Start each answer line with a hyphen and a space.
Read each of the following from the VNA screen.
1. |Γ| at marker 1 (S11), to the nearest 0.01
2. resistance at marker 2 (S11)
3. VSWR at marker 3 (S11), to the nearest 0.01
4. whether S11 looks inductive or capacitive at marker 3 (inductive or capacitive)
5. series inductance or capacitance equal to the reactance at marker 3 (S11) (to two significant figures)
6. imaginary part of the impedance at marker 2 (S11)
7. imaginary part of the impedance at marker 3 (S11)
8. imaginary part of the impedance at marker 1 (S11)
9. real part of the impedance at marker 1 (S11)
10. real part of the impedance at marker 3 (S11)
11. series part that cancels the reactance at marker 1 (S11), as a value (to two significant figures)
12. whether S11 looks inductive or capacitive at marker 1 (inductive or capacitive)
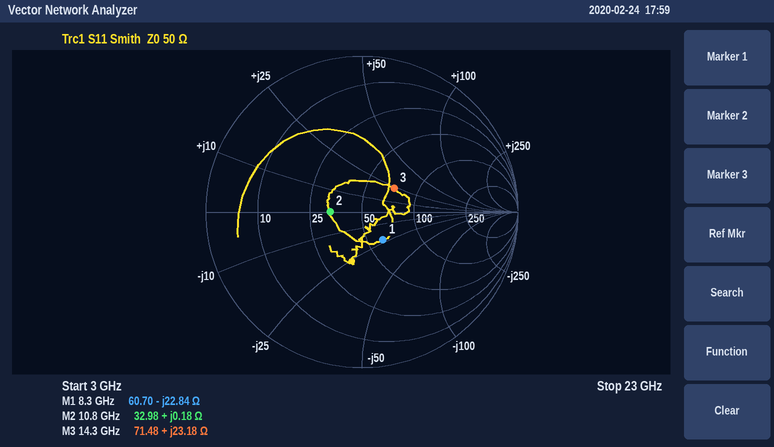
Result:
- 0.22
- 32.98 Ω
- 1.69
- inductive
- 260 pH
- +0.18 Ω
- +23.18 Ω
- -22.84 Ω
- 60.70 Ω
- 71.48 Ω
- 440 pH
- capacitive
